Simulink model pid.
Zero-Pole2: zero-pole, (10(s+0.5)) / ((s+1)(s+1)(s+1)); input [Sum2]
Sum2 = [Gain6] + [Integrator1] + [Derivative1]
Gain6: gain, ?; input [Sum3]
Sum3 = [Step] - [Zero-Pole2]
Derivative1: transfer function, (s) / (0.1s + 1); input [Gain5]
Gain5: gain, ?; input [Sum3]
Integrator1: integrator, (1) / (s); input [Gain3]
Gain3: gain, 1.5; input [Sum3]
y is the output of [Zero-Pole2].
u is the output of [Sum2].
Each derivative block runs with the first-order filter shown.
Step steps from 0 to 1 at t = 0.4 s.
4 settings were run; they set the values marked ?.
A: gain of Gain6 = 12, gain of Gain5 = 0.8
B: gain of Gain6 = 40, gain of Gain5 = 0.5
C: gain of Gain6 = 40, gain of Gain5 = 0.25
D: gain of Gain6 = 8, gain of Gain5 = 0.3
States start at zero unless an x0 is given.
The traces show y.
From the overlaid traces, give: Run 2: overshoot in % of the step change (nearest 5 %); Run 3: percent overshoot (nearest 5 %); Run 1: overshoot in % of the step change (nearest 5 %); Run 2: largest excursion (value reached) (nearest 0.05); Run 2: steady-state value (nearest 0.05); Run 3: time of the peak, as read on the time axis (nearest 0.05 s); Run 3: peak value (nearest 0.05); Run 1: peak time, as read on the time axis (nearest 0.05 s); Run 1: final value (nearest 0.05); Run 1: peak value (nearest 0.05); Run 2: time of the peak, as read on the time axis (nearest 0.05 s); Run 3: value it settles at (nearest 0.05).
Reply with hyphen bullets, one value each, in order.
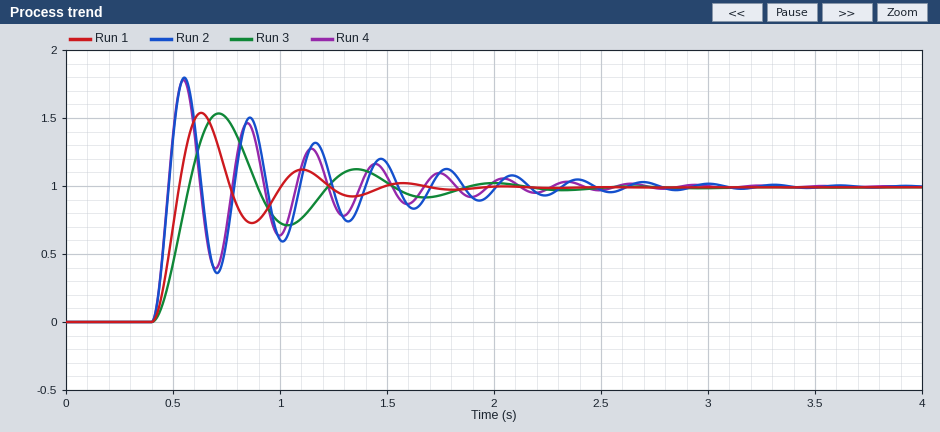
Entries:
- 80 %
- 55 %
- 55 %
- 1.80
- 1.00
- 0.70 s
- 1.55
- 0.65 s
- 1.00
- 1.55
- 0.55 s
- 1.00
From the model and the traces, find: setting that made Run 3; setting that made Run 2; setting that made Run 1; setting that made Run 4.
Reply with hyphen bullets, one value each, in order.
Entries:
- D
- C
- A
- B
